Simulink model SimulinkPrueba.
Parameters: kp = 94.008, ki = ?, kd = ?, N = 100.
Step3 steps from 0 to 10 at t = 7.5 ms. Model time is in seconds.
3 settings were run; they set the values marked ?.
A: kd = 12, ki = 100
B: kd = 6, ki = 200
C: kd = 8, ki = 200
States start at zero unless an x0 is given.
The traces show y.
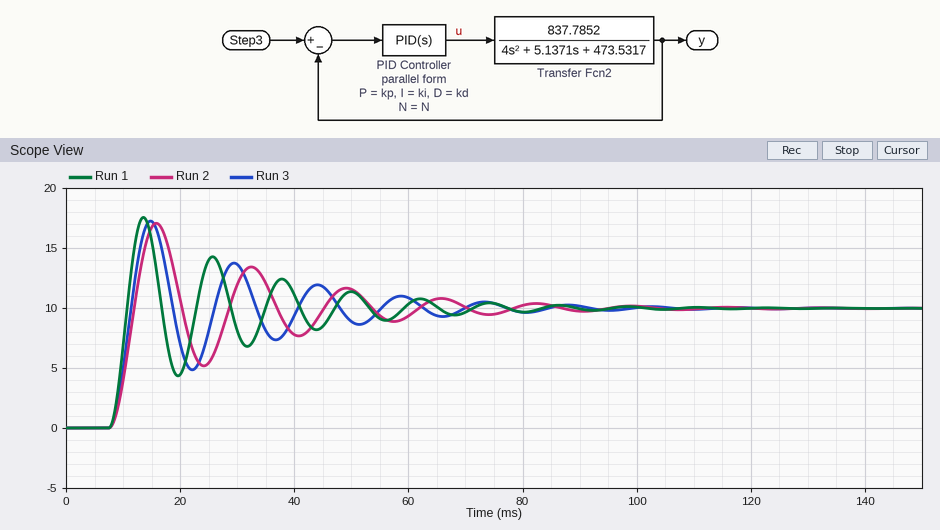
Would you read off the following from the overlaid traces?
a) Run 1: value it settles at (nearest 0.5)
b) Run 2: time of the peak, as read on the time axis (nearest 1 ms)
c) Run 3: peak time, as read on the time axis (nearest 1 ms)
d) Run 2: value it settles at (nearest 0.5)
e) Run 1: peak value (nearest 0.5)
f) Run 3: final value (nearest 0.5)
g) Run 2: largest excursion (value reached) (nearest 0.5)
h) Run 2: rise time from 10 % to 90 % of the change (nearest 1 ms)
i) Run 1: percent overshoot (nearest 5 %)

10.0
16 ms
15 ms
10.0
17.5
10.0
17.0
3 ms
75 %
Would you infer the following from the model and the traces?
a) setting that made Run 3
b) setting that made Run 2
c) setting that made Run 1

C
B
A
